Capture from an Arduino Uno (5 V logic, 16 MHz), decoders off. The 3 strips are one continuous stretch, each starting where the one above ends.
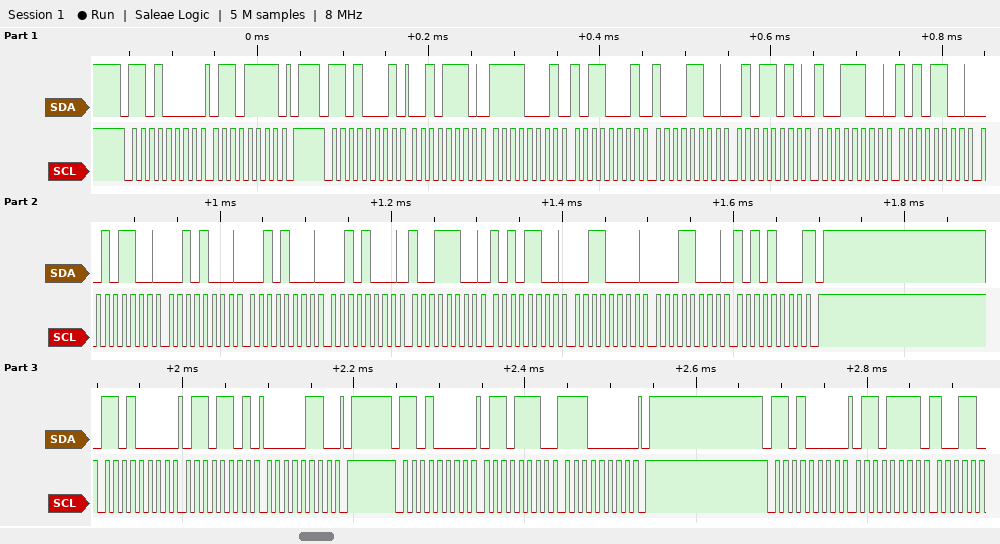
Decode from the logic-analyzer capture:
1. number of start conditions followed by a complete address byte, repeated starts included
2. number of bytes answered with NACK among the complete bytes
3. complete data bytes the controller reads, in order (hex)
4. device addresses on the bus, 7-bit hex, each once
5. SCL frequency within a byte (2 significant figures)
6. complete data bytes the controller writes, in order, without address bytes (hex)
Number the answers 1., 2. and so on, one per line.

1. 5
2. 1
3. 2E F1 B1 8C 5A 9C AC 2C 28 28 28 9C AC 30 18 A8
4. 0x68
5. 100 kHz
6. 6F 6D 06 6E E0 6F
